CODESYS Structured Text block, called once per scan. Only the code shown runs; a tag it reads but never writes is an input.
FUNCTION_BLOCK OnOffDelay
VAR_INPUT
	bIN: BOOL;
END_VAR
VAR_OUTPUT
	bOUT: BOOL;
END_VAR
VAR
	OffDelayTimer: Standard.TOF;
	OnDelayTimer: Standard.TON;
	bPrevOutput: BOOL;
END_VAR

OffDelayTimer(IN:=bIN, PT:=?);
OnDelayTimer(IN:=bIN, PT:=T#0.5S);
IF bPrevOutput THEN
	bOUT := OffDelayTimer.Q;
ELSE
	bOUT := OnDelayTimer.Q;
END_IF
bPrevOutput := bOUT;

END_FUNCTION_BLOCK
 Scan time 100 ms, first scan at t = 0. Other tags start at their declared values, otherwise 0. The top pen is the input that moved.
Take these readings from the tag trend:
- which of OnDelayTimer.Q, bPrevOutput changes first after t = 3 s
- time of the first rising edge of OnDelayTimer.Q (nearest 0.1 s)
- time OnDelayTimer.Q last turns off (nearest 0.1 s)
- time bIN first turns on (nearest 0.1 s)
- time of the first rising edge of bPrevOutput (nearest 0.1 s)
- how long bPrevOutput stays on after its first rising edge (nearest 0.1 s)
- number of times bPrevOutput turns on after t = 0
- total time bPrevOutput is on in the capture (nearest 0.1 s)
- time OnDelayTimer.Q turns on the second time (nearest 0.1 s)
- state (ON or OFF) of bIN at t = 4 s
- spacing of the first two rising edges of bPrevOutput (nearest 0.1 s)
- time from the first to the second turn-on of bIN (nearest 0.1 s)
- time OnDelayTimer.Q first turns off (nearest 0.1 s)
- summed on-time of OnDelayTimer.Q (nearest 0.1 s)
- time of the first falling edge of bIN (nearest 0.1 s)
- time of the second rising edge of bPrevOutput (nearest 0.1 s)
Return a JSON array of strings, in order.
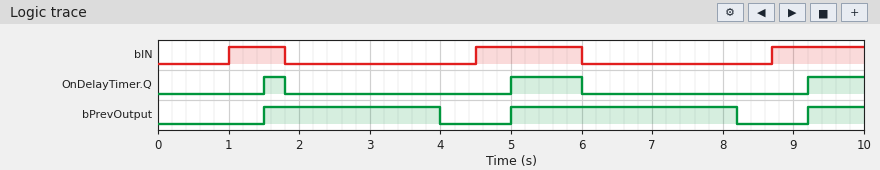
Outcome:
["bPrevOutput", "1.5 s", "6.0 s", "1.0 s", "1.5 s", "2.5 s", "3", "6.5 s", "5.0 s", "OFF", "3.5 s", "3.5 s", "1.8 s", "2.1 s", "1.8 s", "5.0 s"]
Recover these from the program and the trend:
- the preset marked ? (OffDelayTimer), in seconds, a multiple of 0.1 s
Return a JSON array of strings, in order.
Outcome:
["2.2 s"]
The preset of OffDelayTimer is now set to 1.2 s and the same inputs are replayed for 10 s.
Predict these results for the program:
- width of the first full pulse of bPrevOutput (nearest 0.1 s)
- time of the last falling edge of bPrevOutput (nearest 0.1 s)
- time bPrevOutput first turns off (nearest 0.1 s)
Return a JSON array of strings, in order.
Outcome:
["1.5 s", "7.2 s", "3.0 s"]
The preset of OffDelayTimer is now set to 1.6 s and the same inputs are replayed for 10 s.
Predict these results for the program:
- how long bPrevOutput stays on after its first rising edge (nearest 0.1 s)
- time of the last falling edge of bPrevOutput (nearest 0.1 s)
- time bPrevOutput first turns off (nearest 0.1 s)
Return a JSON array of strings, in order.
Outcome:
["1.9 s", "7.6 s", "3.4 s"]
